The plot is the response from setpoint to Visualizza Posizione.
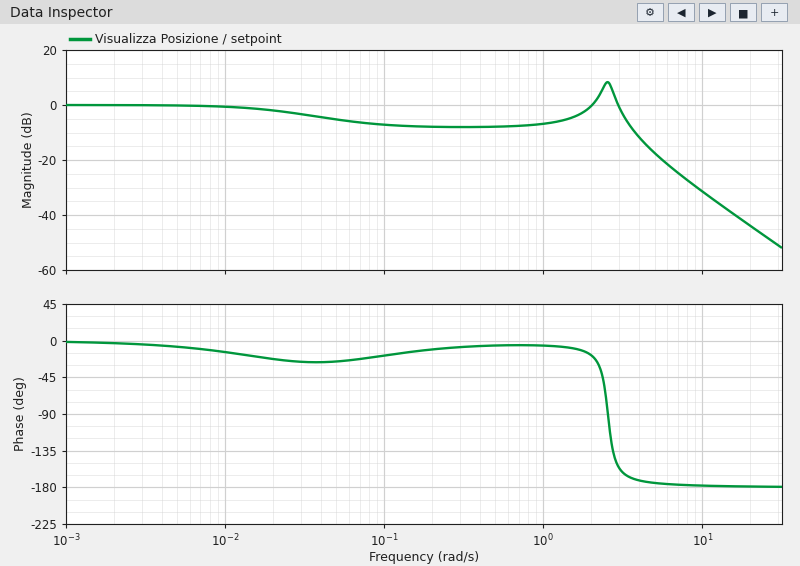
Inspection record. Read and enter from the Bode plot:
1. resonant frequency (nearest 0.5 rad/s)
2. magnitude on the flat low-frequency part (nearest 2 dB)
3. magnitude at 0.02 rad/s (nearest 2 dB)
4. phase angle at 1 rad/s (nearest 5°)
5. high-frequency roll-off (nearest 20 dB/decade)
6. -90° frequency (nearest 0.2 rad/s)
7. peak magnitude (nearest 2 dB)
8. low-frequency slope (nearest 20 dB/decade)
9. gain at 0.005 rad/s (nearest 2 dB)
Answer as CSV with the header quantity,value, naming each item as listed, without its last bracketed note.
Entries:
quantity,value
resonant frequency,2.5 rad/s
magnitude on the flat low-frequency part,0 dB
magnitude at 0.02 rad/s,-2 dB
phase angle at 1 rad/s,-5°
high-frequency roll-off,-40 dB/decade
-90° frequency,2.6 rad/s
peak magnitude,8 dB
low-frequency slope,0 dB/decade
gain at 0.005 rad/s,0 dB
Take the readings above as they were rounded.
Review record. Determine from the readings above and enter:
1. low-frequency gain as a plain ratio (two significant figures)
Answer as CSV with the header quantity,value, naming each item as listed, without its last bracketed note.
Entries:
quantity,value
low-frequency gain as a plain ratio,1.0
